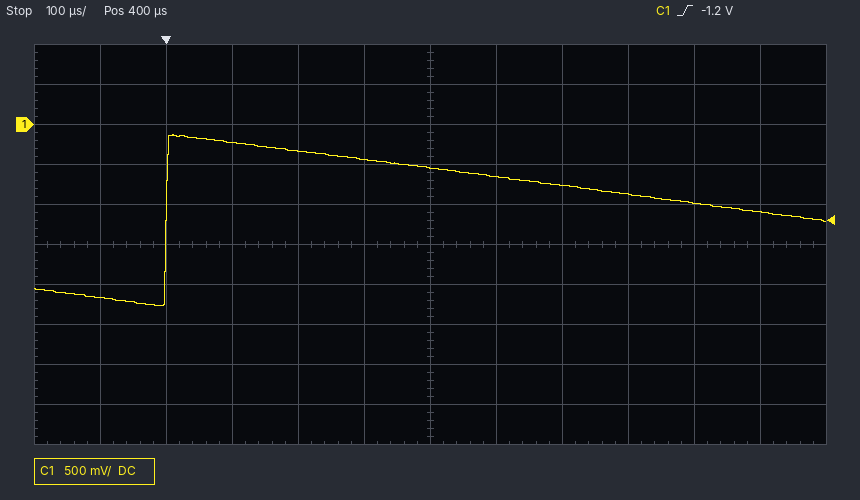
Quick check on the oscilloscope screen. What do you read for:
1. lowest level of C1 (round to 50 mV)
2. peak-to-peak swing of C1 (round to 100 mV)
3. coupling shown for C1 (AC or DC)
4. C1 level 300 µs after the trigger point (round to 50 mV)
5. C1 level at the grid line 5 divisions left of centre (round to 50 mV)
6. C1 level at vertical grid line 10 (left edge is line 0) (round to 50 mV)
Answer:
-2.25 V
2.10 V
DC
-450 mV
-2.15 V
-1.00 V
